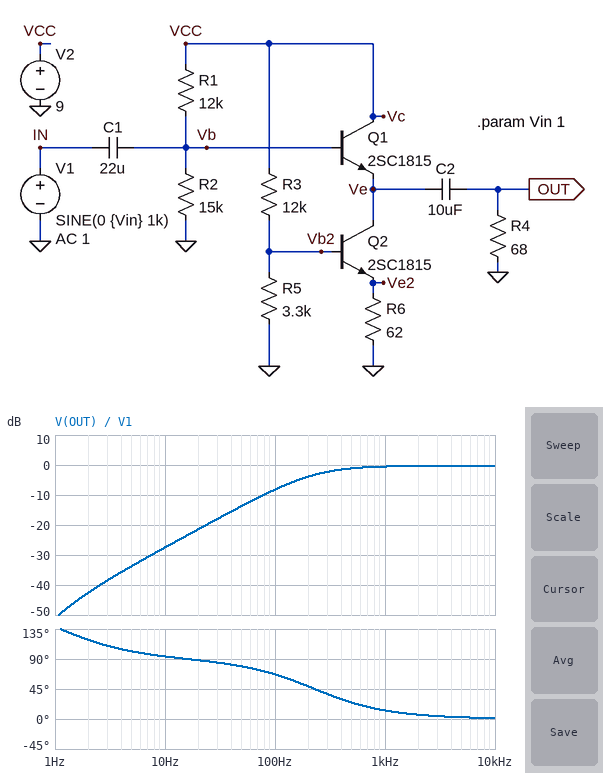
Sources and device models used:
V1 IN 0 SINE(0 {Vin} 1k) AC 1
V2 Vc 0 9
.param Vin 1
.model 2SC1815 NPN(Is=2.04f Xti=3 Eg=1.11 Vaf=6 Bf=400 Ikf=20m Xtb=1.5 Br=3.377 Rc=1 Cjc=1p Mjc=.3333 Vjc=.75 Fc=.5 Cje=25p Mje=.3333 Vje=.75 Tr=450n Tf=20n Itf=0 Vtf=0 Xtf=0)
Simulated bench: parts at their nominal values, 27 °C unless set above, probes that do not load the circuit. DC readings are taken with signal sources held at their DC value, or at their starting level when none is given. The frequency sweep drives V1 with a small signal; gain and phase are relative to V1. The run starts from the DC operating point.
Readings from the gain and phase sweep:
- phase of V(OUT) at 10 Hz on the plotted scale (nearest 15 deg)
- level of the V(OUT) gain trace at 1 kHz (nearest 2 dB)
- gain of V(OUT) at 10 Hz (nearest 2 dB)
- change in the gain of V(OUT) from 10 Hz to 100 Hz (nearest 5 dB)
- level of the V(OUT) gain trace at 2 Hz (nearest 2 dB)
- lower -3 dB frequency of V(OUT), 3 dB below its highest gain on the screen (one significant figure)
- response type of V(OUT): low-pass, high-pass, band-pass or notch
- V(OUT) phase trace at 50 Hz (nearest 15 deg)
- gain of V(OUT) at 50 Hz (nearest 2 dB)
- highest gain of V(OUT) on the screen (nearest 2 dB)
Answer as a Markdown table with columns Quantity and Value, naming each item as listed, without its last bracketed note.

| Quantity | Value |
|---|---|
| phase of V(OUT) at 10 Hz on the plotted scale | 90 deg |
| level of the V(OUT) gain trace at 1 kHz | 0 dB |
| gain of V(OUT) at 10 Hz | -28 dB |
| change in the gain of V(OUT) from 10 Hz to 100 Hz | 20 dB |
| level of the V(OUT) gain trace at 2 Hz | -42 dB |
| lower -3 dB frequency of V(OUT), 3 dB below its highest gain on the screen | 200 Hz |
| response type of V(OUT): low-pass, high-pass, band-pass or notch | high-pass |
| V(OUT) phase trace at 50 Hz | 75 deg |
| gain of V(OUT) at 50 Hz | -14 dB |
| highest gain of V(OUT) on the screen | 0 dB |
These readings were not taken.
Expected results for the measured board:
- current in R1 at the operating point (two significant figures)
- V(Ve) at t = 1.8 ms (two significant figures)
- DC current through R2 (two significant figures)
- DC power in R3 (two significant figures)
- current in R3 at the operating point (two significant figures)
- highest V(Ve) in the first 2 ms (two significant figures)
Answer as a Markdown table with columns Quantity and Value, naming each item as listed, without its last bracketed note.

| Quantity | Value |
|---|---|
| current in R1 at the operating point | 350 µA |
| V(Ve) at t = 1.8 ms | 3.1 V |
| DC current through R2 | 320 µA |
| DC power in R3 | 4.3 mW |
| current in R3 at the operating point | 600 µA |
| highest V(Ve) in the first 2 ms | 5.0 V |
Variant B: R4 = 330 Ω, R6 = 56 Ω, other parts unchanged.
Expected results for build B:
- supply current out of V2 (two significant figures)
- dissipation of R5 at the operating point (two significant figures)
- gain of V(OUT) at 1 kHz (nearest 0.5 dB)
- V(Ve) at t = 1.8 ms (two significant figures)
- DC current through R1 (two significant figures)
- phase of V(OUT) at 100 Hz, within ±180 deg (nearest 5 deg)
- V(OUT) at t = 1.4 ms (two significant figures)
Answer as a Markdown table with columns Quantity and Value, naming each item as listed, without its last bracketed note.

| Quantity | Value |
|---|---|
| supply current out of V2 | 19 mA |
| dissipation of R5 at the operating point | 980 µW |
| gain of V(OUT) at 1 kHz | 0 dB |
| V(Ve) at t = 1.8 ms | 3.0 V |
| DC current through R1 | 360 µA |
| phase of V(OUT) at 100 Hz, within ±180 deg | 25 deg |
| V(OUT) at t = 1.4 ms | 510 mV |
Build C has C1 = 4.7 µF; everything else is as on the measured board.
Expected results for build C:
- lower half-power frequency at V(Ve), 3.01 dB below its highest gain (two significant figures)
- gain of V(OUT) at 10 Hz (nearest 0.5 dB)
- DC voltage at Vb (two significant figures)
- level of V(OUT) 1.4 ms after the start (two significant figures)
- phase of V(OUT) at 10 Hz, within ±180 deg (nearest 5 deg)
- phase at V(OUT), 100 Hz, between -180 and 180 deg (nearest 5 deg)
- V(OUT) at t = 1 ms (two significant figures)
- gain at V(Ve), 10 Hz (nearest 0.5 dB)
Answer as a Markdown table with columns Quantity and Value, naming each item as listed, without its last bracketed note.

| Quantity | Value |
|---|---|
| lower half-power frequency at V(Ve), 3.01 dB below its highest gain | 5.2 Hz |
| gain of V(OUT) at 10 Hz | -28.5 dB |
| DC voltage at Vb | 4.8 V |
| level of V(OUT) 1.4 ms after the start | 330 mV |
| phase of V(OUT) at 10 Hz, within ±180 deg | 115 deg |
| phase at V(OUT), 100 Hz, between -180 and 180 deg | 70 deg |
| V(OUT) at t = 1 ms | 160 mV |
| gain at V(Ve), 10 Hz | -1.0 dB |
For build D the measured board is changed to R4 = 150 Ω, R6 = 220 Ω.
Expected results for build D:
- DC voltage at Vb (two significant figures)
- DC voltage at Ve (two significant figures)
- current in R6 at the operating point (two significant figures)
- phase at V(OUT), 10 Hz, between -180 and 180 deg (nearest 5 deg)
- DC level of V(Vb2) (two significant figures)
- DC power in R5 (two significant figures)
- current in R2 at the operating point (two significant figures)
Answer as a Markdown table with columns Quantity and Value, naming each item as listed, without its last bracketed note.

| Quantity | Value |
|---|---|
| DC voltage at Vb | 4.9 V |
| DC voltage at Ve | 4.2 V |
| current in R6 at the operating point | 5.3 mA |
| phase at V(OUT), 10 Hz, between -180 and 180 deg | 90 deg |
| DC level of V(Vb2) | 1.9 V |
| DC power in R5 | 1.1 mW |
| current in R2 at the operating point | 330 µA |
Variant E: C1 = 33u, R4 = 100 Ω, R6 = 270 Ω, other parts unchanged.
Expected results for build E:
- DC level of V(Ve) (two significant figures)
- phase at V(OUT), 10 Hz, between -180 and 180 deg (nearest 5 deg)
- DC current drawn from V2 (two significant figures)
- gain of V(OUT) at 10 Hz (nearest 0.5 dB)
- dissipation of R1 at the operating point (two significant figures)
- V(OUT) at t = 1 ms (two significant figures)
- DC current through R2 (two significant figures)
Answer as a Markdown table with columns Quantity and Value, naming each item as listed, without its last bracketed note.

| Quantity | Value |
|---|---|
| DC level of V(Ve) | 4.2 V |
| phase at V(OUT), 10 Hz, between -180 and 180 deg | 90 deg |
| DC current drawn from V2 | 5.3 mA |
| gain of V(OUT) at 10 Hz | -24.0 dB |
| dissipation of R1 at the operating point | 1.4 mW |
| V(OUT) at t = 1 ms | -38 mV |
| DC current through R2 | 330 µA |
